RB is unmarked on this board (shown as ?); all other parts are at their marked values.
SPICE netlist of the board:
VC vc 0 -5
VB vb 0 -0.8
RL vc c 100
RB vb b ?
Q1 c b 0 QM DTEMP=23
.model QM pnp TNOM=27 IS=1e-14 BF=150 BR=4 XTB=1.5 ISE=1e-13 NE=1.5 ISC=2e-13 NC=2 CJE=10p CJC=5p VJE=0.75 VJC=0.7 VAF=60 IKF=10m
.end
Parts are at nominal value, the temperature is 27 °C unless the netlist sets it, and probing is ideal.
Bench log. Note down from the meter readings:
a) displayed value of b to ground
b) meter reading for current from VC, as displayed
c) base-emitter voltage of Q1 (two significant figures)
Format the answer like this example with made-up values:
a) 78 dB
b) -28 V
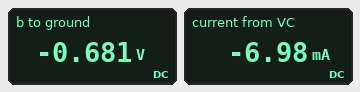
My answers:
a) -0.681 V
b) -6.98 mA
c) -680 mV
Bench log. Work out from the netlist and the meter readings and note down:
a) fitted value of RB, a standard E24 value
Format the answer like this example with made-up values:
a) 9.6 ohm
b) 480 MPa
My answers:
a) 1.6 kΩ
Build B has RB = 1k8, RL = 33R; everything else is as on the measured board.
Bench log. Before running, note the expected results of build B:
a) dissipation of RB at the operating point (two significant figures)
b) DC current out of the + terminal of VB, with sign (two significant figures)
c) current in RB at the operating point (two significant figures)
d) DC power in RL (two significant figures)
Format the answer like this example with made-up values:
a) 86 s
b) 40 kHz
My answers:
a) 8.3 µW
b) -68 µA
c) 68 µA
d) 1.4 mW
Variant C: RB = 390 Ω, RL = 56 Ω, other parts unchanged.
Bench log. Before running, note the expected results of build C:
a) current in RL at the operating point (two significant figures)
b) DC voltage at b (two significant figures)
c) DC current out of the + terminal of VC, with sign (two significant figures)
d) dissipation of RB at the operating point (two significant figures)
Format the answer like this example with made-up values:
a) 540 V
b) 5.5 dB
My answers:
a) 15 mA
b) -710 mV
c) -15 mA
d) 20 µW
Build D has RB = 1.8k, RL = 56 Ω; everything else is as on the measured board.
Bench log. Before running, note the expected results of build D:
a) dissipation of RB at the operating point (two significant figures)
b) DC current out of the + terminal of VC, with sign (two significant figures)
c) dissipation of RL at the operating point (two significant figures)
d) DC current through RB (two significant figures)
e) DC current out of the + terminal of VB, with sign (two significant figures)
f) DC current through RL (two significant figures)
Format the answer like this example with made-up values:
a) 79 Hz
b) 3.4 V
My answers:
a) 8.3 µW
b) -6.5 mA
c) 2.4 mW
d) 68 µA
e) -68 µA
f) 6.5 mA
